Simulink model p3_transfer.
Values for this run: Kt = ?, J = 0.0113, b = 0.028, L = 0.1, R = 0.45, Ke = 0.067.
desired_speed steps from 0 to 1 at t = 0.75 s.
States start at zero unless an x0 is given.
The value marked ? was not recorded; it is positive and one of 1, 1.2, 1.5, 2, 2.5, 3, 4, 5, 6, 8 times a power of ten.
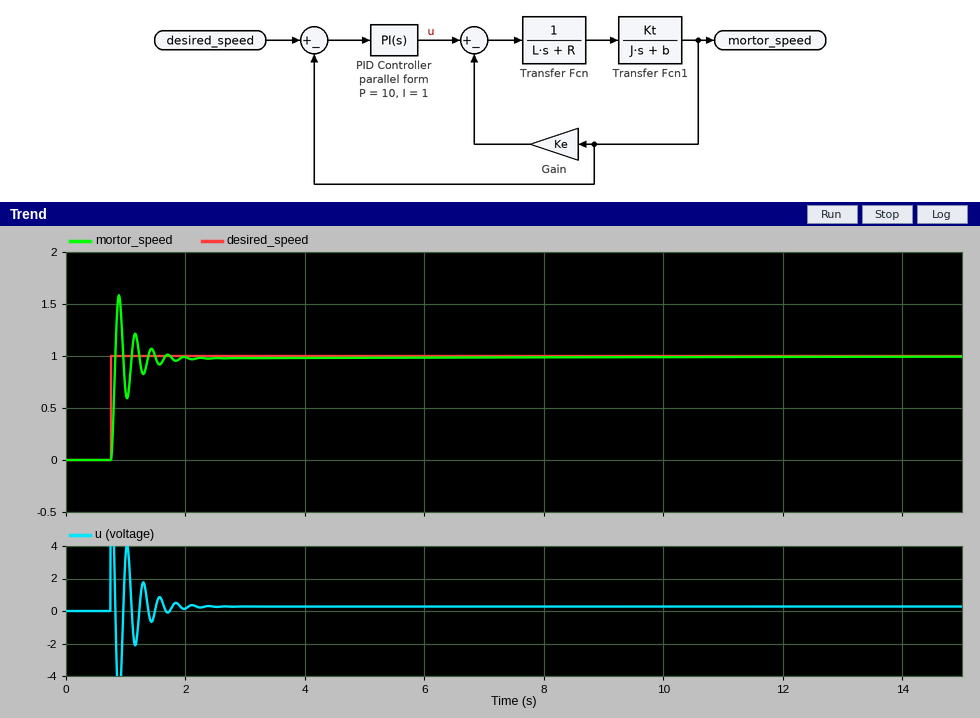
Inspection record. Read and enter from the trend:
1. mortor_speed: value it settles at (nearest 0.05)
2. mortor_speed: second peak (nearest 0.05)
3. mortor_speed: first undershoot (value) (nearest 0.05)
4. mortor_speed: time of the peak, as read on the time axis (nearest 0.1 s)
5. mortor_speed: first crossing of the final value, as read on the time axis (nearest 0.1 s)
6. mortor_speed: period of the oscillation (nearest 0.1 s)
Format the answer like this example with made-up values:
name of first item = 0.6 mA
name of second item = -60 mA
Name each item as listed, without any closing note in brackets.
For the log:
mortor_speed: value it settles at = 1.00
mortor_speed: second peak = 1.20
mortor_speed: first undershoot (value) = 0.60
mortor_speed: time of the peak, as read on the time axis = 0.9 s
mortor_speed: first crossing of the final value, as read on the time axis = 0.8 s
mortor_speed: period of the oscillation = 0.3 s
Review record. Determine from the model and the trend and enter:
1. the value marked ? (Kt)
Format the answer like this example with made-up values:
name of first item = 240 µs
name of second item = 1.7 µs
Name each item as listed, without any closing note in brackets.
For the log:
the value marked ? = 0.06
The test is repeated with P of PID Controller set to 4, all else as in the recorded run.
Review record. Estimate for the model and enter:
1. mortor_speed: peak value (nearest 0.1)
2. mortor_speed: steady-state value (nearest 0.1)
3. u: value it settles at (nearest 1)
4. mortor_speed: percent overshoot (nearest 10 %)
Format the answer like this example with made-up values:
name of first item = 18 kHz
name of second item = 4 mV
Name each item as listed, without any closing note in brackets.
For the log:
mortor_speed: peak value = 1.4
mortor_speed: steady-state value = 1.0
u: value it settles at = 0
mortor_speed: percent overshoot = 40 %
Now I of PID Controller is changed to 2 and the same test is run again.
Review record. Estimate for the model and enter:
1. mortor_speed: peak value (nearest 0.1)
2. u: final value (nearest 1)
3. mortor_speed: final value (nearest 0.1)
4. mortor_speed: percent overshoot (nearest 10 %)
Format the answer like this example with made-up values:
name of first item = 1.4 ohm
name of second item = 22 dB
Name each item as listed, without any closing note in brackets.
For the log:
mortor_speed: peak value = 1.6
u: final value = 0
mortor_speed: final value = 1.0
mortor_speed: percent overshoot = 60 %
